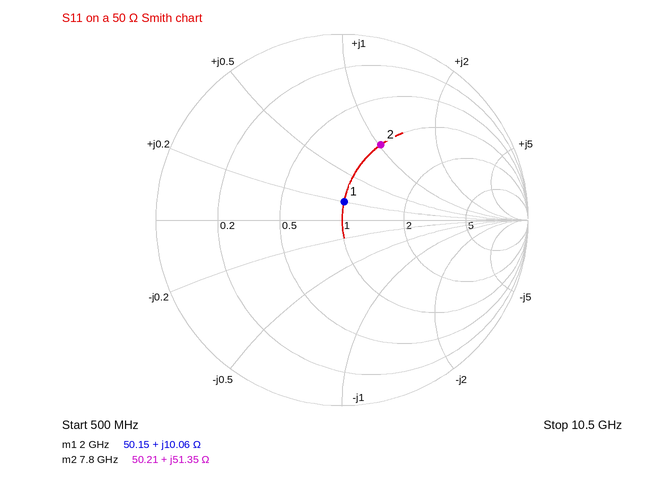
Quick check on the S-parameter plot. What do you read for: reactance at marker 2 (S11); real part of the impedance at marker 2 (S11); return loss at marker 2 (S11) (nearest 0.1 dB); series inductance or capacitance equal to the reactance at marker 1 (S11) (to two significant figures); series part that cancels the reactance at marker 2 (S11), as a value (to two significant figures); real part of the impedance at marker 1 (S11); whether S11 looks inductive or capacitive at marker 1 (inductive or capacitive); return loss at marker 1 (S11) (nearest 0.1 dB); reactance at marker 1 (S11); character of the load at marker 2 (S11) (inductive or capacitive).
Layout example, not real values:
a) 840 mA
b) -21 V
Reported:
a) +51.35 Ω
b) 50.21 Ω
c) 6.8 dB
d) 800 pH
e) 400 fF
f) 50.15 Ω
g) inductive
h) 20.0 dB
i) +10.06 Ω
j) inductive
